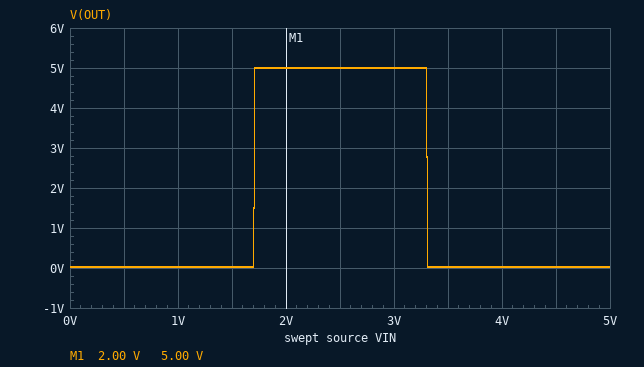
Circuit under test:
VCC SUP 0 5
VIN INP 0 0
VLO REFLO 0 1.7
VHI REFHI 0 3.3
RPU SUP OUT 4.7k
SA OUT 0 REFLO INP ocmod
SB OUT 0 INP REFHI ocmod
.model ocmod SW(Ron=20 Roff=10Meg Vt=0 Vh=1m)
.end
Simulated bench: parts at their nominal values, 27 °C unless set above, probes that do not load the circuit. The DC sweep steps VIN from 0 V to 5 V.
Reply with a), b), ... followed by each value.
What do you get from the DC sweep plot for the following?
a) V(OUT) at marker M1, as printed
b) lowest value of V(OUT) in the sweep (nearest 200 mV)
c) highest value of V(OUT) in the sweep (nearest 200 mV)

a) 5.00 V
b) 0 V
c) 5.0 V
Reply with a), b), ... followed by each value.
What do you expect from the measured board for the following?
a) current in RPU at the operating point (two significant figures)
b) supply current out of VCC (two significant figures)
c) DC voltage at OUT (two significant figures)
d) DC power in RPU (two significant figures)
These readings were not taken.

a) 1.1 mA
b) 1.1 mA
c) 21 mV
d) 5.3 mW
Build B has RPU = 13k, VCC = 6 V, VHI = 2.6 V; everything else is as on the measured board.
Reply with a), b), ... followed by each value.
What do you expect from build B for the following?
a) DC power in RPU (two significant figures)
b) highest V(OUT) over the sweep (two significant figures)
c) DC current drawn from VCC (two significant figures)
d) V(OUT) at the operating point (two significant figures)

a) 2.8 mW
b) 6.0 V
c) 460 µA
d) 9.2 mV
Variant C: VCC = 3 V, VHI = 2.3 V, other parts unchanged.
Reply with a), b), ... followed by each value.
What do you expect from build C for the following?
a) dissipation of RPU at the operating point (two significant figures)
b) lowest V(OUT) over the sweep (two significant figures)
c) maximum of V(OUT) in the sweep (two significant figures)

a) 1.9 mW
b) 13 mV
c) 3.0 V
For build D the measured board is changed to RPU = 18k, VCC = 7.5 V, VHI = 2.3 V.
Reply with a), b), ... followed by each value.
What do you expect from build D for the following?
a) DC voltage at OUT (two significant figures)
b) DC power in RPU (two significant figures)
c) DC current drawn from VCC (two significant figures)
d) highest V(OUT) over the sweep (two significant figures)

a) 8.3 mV
b) 3.1 mW
c) 420 µA
d) 7.5 V
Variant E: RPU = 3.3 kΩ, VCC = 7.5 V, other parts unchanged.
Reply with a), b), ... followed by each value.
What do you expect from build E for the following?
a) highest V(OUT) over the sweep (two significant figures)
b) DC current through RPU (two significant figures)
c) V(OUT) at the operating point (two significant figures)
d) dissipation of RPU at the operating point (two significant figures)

a) 7.5 V
b) 2.3 mA
c) 45 mV
d) 17 mW
